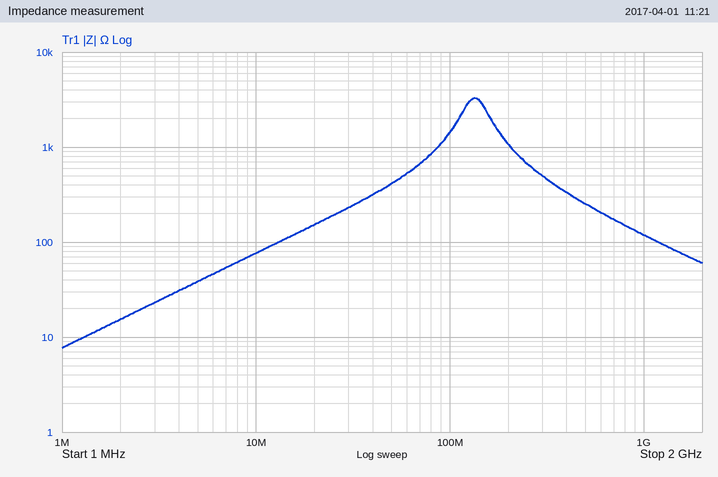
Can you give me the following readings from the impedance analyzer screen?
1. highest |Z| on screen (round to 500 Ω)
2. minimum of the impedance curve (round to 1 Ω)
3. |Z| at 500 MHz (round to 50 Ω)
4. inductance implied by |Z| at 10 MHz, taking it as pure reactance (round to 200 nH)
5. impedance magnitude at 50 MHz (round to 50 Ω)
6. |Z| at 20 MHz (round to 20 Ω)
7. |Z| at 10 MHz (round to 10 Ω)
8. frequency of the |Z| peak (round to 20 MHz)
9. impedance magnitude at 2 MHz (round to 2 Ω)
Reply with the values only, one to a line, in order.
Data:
3.5 kΩ
8 Ω
250 Ω
1.2 µH
400 Ω
160 Ω
80 Ω
140 MHz
16 Ω
